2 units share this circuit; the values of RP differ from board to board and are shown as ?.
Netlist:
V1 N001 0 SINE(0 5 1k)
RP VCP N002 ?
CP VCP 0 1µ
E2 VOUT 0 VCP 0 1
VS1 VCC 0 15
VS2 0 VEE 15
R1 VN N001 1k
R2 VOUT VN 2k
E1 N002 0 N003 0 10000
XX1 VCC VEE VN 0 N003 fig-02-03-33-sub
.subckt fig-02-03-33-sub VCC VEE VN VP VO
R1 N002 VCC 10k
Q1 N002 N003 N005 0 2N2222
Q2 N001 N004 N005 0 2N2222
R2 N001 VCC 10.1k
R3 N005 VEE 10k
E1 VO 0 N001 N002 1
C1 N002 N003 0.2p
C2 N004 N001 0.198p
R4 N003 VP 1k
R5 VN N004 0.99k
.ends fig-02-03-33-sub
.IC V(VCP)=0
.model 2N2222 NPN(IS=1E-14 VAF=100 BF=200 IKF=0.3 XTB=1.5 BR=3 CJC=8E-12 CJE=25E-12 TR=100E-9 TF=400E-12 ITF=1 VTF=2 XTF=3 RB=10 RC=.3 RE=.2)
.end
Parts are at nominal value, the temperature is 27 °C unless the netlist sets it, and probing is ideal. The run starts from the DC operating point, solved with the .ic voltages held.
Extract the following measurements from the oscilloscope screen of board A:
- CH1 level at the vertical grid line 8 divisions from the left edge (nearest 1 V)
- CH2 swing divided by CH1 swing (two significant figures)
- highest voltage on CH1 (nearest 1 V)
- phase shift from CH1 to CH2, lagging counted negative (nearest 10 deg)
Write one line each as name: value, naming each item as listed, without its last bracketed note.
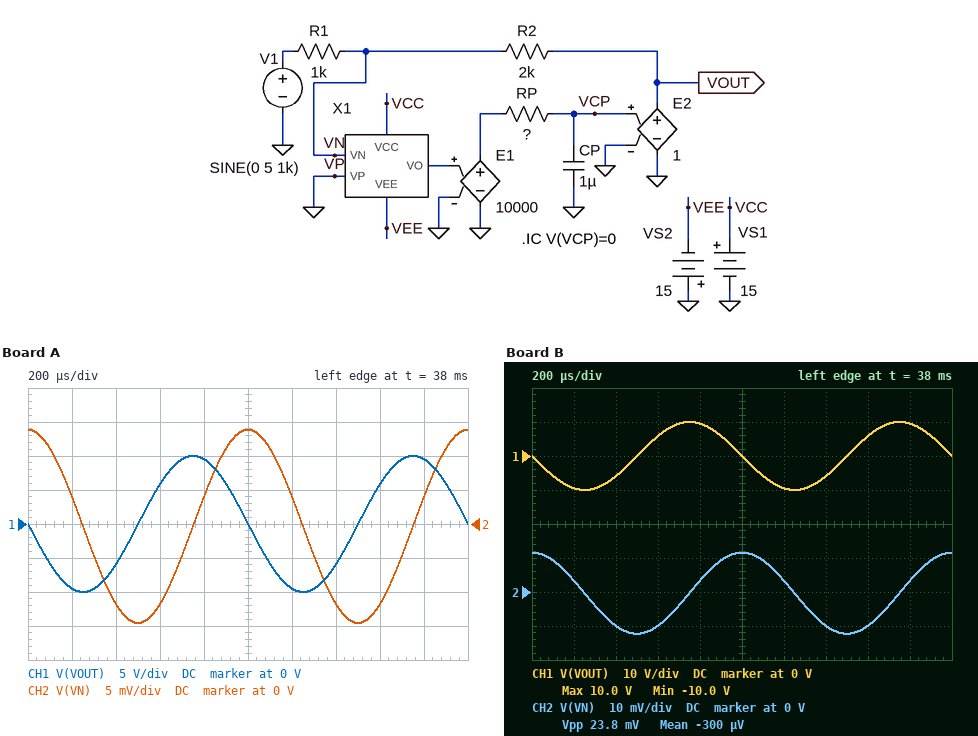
CH1 level at the vertical grid line 8 divisions from the left edge: 6 V
CH2 swing divided by CH1 swing: 0.0014
highest voltage on CH1: 10 V
phase shift from CH1 to CH2, lagging counted negative: -90 deg
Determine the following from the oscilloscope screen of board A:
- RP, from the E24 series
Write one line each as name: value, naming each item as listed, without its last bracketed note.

RP, from the E24 series: 510 kΩ
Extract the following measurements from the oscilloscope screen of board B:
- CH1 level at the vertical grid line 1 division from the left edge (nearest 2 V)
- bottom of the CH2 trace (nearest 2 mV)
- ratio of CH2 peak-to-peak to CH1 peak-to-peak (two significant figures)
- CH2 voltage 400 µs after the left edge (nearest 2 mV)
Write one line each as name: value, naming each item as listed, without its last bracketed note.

CH1 level at the vertical grid line 1 division from the left edge: -10 V
bottom of the CH2 trace: -12 mV
ratio of CH2 peak-to-peak to CH1 peak-to-peak: 0.0012
CH2 voltage 400 µs after the left edge: -10 mV
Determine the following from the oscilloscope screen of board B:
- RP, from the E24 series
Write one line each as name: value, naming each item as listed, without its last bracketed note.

RP, from the E24 series: 430 kΩ
